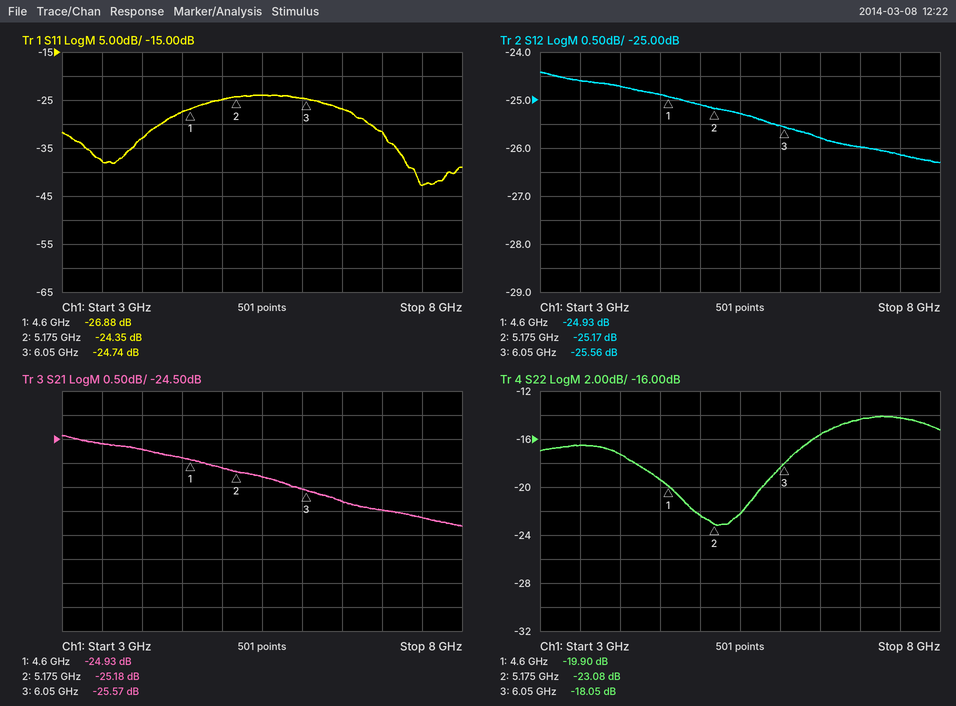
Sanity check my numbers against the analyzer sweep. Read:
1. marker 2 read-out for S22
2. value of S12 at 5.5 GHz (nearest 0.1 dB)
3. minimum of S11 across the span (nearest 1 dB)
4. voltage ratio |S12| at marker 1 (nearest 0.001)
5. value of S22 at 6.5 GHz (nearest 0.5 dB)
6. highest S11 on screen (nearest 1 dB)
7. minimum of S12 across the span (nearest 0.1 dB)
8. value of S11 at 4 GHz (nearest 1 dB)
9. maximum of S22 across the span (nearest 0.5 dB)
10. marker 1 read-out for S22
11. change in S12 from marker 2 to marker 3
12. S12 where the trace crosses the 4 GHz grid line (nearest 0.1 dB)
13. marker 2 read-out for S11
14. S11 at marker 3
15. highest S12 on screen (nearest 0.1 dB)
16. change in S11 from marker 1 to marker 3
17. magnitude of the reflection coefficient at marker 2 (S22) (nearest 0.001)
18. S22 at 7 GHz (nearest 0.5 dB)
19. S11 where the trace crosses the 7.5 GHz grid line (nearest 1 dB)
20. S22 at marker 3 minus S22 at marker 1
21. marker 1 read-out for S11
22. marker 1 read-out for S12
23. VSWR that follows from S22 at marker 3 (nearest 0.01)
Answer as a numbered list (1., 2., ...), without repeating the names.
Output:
1. -23.08 dB
2. -25.3 dB
3. -43 dB
4. 0.057
5. -15.5 dB
6. -24 dB
7. -26.3 dB
8. -33 dB
9. -14.0 dB
10. -19.90 dB
11. -0.39 dB
12. -24.7 dB
13. -24.35 dB
14. -24.74 dB
15. -24.4 dB
16. 2.14 dB
17. 0.070
18. -14.5 dB
19. -43 dB
20. 1.85 dB
21. -26.88 dB
22. -24.93 dB
23. 1.29
